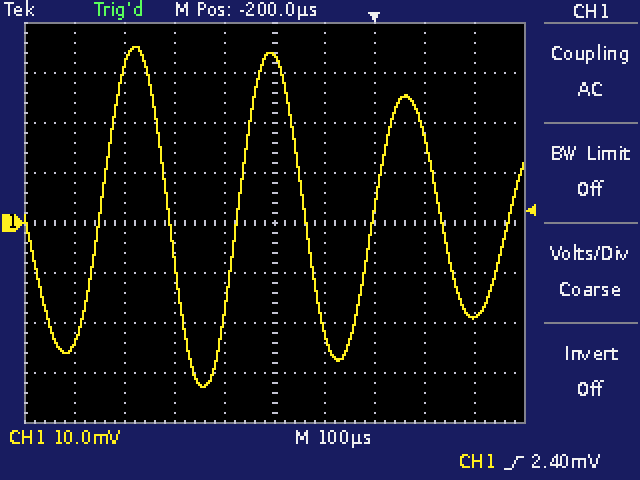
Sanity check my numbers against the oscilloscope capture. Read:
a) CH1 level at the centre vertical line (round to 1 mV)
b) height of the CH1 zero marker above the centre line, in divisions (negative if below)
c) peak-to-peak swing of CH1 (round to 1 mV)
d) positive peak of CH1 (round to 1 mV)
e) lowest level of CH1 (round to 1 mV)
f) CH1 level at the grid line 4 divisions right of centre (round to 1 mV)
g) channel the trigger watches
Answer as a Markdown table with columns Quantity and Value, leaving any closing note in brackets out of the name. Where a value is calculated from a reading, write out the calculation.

| Quantity | Value |
|---|---|
| CH1 level at the centre vertical line | 33 mV |
| height of the CH1 zero marker above the centre line, in divisions | 0.0 div |
| peak-to-peak swing of CH1 | 35 mV − (-33 mV) = 68 mV |
| positive peak of CH1 | 35 mV |
| lowest level of CH1 | -33 mV |
| CH1 level at the grid line 4 divisions right of centre | -19 mV |
| channel the trigger watches | CH1 |
